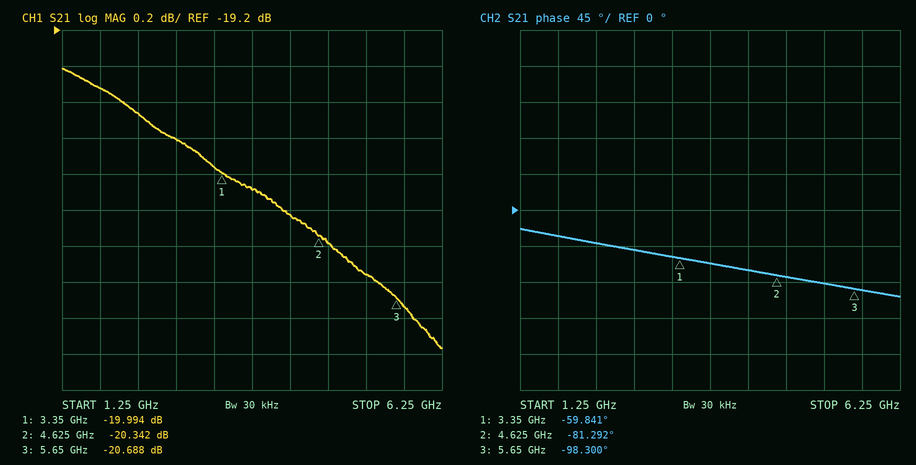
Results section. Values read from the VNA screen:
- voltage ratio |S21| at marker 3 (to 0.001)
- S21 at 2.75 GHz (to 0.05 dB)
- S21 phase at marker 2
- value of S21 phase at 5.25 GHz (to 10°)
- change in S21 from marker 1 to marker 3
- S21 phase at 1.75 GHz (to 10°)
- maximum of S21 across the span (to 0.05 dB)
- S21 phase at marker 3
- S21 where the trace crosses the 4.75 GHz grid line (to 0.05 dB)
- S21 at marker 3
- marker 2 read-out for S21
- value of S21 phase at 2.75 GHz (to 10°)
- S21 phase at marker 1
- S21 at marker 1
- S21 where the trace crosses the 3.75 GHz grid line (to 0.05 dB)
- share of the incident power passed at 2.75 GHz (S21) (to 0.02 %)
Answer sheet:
0.092
-19.80 dB
-81.292°
-90°
-0.694 dB
-30°
-19.40 dB
-98.300°
-20.40 dB
-20.688 dB
-20.342 dB
-50°
-59.841°
-19.994 dB
-20.10 dB
1.04 %
